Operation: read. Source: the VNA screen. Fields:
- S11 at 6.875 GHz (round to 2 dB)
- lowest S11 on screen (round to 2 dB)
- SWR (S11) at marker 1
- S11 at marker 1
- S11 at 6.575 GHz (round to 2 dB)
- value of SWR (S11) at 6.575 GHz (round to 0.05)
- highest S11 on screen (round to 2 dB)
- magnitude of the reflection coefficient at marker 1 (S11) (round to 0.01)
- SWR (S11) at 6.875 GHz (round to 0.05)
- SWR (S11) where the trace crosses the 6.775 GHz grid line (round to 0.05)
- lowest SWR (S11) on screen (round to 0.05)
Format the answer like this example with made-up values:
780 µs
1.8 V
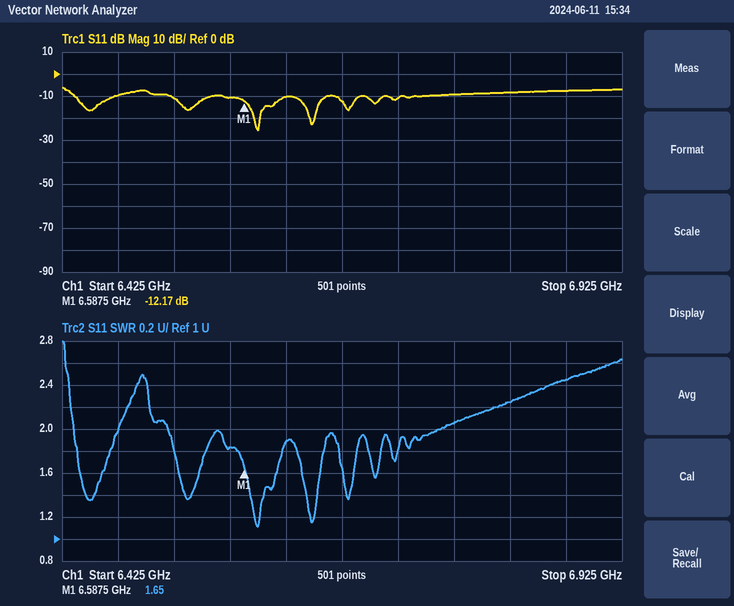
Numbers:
-8 dB
-26 dB
1.65
-12.17 dB
-10 dB
1.85
-6 dB
0.25
2.45
2.05
1.10
